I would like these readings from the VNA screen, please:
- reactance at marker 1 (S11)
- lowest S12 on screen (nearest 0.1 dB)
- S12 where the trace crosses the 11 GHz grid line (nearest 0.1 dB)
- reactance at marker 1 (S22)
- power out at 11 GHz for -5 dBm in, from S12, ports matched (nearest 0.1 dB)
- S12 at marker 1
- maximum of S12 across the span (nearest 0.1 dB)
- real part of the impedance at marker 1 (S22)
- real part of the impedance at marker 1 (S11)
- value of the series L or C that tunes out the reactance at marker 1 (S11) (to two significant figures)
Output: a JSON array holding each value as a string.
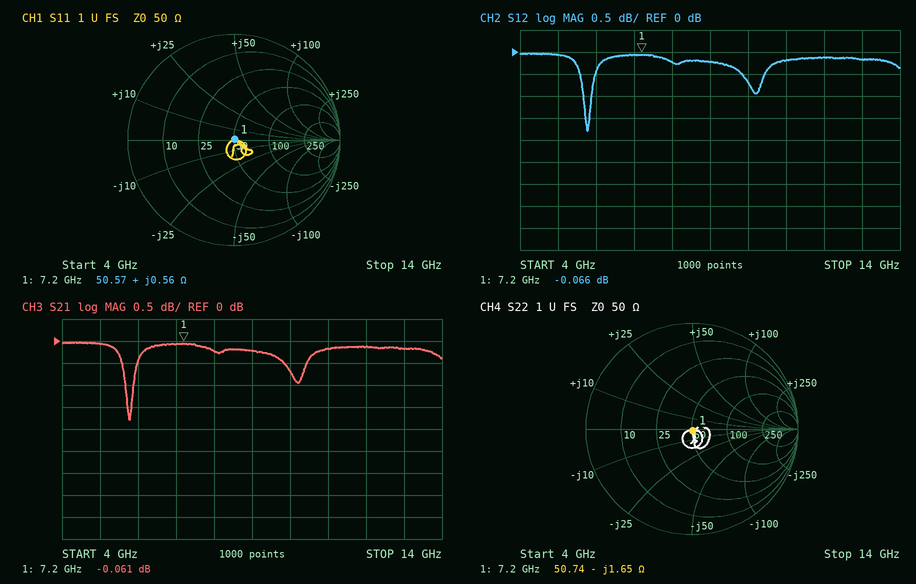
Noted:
["+0.56 Ω", "-1.8 dB", "-0.2 dB", "-1.65 Ω", "-5.2 dBm", "-0.066 dB", "0.0 dB", "50.74 Ω", "50.57 Ω", "39 pF"]
